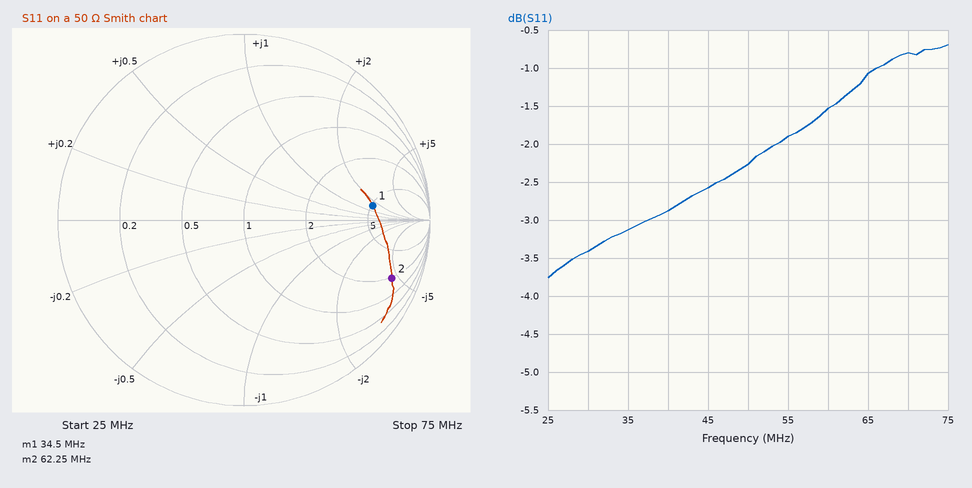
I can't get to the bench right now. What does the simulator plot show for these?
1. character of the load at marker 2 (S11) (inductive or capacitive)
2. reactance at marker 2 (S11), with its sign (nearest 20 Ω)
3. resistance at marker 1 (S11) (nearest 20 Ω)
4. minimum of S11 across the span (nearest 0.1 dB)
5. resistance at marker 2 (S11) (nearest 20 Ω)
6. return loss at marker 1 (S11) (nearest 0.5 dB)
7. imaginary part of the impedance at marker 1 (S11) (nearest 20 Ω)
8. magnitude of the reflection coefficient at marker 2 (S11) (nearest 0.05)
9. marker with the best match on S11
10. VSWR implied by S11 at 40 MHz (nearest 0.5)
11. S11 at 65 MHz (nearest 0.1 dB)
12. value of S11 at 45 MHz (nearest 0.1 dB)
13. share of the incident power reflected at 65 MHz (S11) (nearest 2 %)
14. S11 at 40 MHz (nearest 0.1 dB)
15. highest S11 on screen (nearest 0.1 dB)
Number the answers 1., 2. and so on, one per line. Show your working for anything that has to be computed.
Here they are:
1. capacitive
2. -220 Ω
3. 260 Ω
4. -3.8 dB
5. 100 Ω
6. 3.0 dB
7. +80 Ω
8. 0.85
9. marker 1
10. |Γ| = 10^(-2.9/20) = 0.7161; VSWR = (1 + 0.7161)/(1 − 0.7161) ≈ 6.0
11. -1.1 dB
12. -2.6 dB
13. 10^(-1.1/10) ≈ 78 %
14. -2.9 dB
15. -0.7 dB
